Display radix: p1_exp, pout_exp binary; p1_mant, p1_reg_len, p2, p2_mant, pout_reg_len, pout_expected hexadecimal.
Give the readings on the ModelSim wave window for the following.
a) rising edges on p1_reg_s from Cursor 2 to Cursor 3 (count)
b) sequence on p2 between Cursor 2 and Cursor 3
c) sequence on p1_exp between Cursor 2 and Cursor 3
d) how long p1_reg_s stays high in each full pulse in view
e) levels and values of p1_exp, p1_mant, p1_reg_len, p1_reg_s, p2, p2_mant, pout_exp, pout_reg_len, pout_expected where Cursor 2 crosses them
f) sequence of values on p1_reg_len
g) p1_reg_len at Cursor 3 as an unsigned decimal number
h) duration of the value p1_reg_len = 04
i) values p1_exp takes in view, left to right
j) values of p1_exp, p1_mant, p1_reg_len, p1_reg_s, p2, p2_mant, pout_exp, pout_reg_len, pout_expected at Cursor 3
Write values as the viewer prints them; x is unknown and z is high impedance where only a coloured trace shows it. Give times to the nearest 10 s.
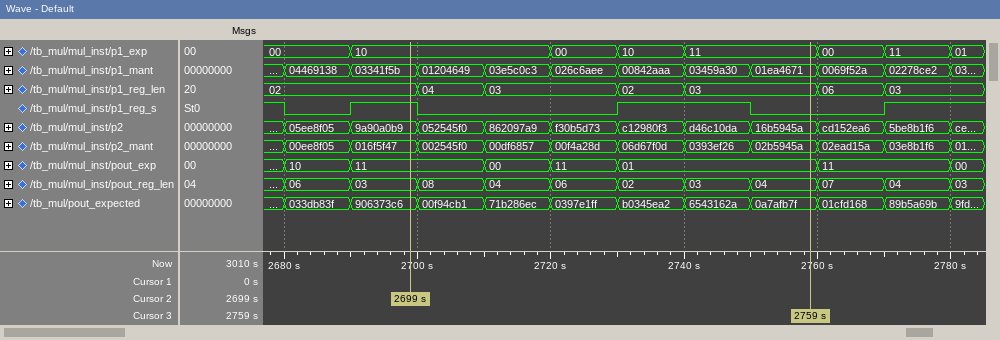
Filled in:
1
9a90a0b9, 052545f0, 862097a9, f30b5d73, c12980f3, d46c10da, 16b5945a
10, 00, 10, 11
10 s, 20 s
p1_exp=10, p1_mant=03341f5b, p1_reg_len=02, p1_reg_s=1, p2=9a90a0b9, p2_mant=016f5f47, pout_exp=11, pout_reg_len=03, pout_expected=906373c6
02, 04, 03, 02, 03, 06, 03
3
10 s
00, 10, 00, 10, 11, 00, 11, 01
p1_exp=11, p1_mant=01ea4671, p1_reg_len=03, p1_reg_s=0, p2=16b5945a, p2_mant=02b5945a, pout_exp=01, pout_reg_len=04, pout_expected=0a7afb7f
